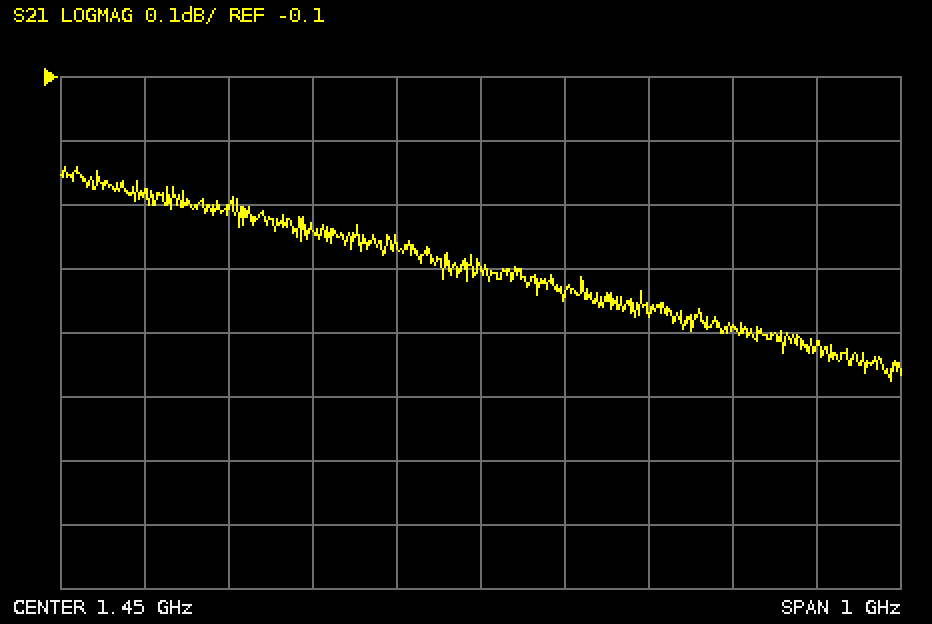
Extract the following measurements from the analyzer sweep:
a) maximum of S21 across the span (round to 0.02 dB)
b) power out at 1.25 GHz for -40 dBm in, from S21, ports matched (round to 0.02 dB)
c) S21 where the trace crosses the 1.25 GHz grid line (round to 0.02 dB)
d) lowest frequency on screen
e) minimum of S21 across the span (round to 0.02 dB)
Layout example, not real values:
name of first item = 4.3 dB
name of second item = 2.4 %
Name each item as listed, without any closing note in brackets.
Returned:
maximum of S21 across the span = -0.24 dB
power out at 1.25 GHz for -40 dBm in, from S21, ports matched = -40.34 dBm
S21 where the trace crosses the 1.25 GHz grid line = -0.34 dB
lowest frequency on screen = 950 MHz
minimum of S21 across the span = -0.58 dB
